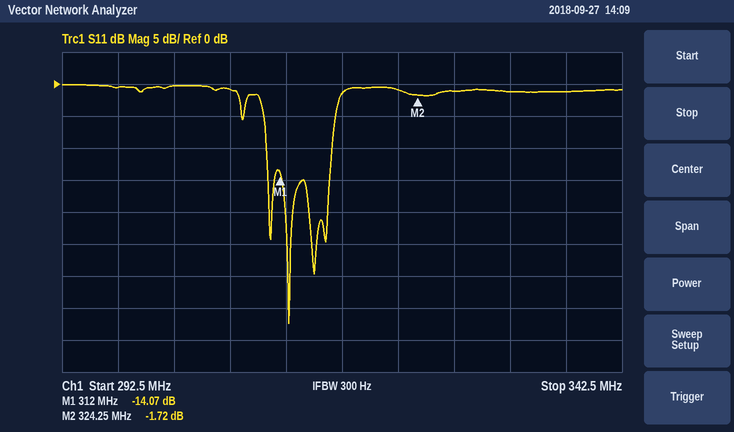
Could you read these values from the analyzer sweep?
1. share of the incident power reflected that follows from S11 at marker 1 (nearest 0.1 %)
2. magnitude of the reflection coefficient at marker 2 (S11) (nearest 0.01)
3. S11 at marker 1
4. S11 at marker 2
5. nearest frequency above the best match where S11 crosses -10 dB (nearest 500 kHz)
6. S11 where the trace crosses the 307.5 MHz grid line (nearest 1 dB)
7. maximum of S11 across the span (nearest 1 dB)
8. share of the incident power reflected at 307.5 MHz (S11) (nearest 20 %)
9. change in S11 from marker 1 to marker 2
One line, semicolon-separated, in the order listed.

3.9 %; 0.82; -14.07 dB; -1.72 dB; 316.5 MHz; -1 dB; 0 dB; 80 %; 12.35 dB
